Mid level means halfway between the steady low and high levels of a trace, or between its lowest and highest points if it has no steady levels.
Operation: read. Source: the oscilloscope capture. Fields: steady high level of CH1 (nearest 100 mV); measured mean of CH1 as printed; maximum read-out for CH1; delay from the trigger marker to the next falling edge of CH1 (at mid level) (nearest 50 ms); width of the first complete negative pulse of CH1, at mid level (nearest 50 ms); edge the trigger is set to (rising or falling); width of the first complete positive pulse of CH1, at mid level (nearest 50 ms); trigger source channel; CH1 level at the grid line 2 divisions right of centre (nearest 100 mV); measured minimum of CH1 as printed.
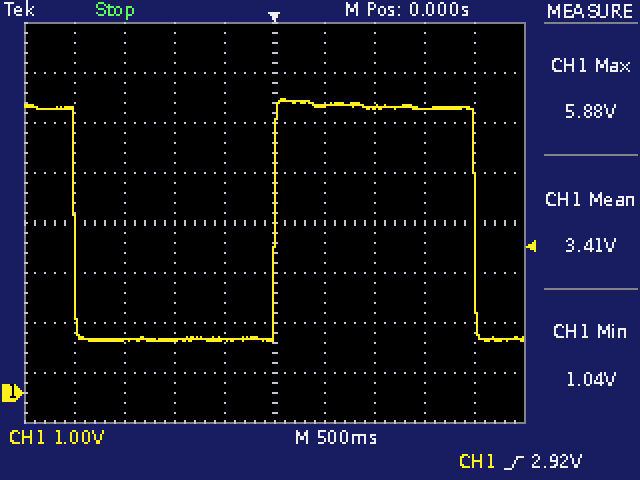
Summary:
5.7 V
3.41 V
5.88 V
2.00 s
2.00 s
rising
2.00 s
CH1
5.7 V
1.04 V
